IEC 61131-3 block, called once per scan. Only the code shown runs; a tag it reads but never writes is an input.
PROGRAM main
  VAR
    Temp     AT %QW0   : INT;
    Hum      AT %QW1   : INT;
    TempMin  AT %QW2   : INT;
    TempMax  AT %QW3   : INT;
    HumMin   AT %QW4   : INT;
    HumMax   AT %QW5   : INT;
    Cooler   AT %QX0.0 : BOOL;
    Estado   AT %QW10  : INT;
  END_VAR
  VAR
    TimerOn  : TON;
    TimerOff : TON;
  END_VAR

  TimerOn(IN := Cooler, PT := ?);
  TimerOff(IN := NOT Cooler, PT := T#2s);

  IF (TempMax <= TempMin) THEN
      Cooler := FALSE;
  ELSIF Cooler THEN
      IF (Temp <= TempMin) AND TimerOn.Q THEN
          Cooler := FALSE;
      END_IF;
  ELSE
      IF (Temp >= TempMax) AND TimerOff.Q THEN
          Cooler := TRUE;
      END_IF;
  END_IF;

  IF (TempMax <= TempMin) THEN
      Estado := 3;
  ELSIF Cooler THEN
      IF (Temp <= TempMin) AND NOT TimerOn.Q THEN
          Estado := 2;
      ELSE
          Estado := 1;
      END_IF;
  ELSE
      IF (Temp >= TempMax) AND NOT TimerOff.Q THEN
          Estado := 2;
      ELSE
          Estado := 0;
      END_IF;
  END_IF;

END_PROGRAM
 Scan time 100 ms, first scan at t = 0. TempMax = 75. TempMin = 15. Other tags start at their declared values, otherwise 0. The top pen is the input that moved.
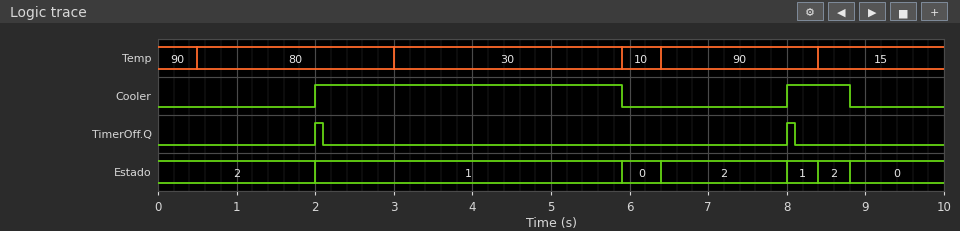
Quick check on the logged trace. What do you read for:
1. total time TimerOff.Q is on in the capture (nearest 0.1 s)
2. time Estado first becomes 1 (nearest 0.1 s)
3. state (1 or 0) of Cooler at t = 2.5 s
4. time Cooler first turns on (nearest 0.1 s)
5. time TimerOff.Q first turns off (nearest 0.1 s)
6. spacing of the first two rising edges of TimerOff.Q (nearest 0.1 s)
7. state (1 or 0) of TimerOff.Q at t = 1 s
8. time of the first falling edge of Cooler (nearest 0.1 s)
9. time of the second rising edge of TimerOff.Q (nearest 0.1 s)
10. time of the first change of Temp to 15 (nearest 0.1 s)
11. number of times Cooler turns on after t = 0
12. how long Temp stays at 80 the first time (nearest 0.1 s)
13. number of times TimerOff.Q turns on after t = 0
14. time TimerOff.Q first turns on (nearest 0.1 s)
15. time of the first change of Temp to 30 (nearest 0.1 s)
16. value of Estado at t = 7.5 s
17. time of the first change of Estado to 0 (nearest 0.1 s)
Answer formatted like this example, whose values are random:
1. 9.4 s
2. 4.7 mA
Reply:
1. 0.2 s
2. 2.0 s
3. 1
4. 2.0 s
5. 2.1 s
6. 6.0 s
7. 0
8. 5.9 s
9. 8.0 s
10. 8.4 s
11. 2
12. 2.5 s
13. 2
14. 2.0 s
15. 3.0 s
16. 2
17. 5.9 s
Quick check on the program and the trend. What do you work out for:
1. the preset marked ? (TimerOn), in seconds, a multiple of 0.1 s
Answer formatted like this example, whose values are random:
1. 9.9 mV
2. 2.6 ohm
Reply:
1. 0.7 s
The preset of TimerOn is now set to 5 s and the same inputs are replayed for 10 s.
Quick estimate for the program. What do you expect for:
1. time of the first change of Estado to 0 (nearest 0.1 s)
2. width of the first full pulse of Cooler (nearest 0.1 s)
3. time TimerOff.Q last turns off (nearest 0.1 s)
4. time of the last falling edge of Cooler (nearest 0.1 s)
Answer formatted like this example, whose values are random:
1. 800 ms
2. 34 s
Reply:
1. 8.4 s
2. 6.4 s
3. 2.1 s
4. 8.4 s
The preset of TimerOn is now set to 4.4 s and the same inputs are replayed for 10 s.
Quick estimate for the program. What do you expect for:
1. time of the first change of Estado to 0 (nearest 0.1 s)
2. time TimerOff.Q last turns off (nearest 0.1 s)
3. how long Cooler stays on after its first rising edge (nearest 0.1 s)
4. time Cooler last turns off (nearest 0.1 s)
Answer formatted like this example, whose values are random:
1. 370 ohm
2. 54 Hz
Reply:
1. 8.4 s
2. 2.1 s
3. 6.4 s
4. 8.4 s
